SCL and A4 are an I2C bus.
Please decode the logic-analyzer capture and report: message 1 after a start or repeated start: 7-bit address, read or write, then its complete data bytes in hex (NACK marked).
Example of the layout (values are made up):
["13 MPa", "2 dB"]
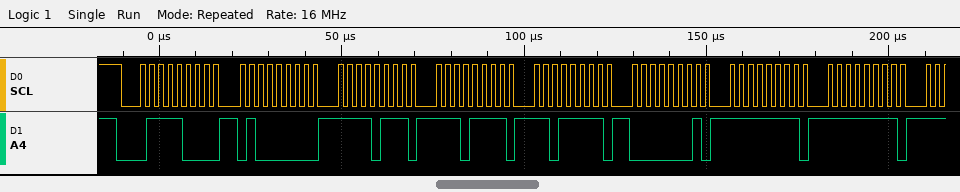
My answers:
["0x3C write: 40 F7 EF DF 01 FF FF"]
